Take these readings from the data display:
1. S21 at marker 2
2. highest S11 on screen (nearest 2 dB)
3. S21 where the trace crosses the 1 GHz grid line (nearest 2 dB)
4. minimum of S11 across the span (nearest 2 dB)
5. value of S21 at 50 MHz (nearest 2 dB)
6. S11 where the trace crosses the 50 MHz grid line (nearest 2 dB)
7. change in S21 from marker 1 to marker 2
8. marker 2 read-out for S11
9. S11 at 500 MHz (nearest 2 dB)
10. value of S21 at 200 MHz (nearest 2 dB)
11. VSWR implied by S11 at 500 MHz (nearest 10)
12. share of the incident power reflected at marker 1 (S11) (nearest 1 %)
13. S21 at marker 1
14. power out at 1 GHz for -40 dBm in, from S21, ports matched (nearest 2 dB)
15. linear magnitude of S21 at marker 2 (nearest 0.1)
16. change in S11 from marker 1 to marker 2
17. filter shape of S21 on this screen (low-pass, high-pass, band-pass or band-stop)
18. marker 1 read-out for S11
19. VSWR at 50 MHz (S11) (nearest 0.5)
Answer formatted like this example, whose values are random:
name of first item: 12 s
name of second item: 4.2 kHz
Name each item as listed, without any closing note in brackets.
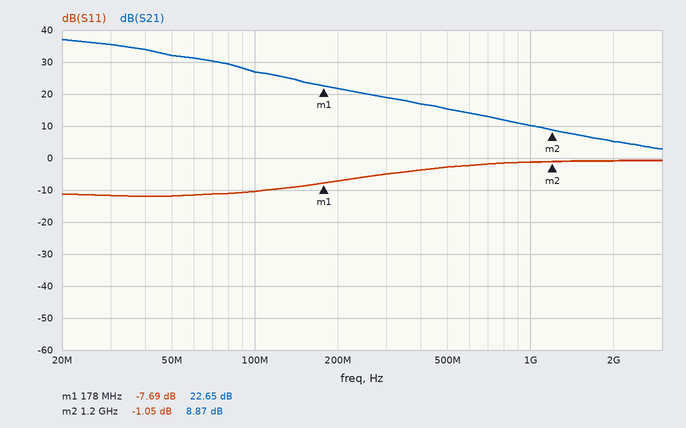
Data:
S21 at marker 2: 8.87 dB
highest S11 on screen: 0 dB
S21 where the trace crosses the 1 GHz grid line: 10 dB
minimum of S11 across the span: -12 dB
value of S21 at 50 MHz: 32 dB
S11 where the trace crosses the 50 MHz grid line: -12 dB
change in S21 from marker 1 to marker 2: -13.78 dB
marker 2 read-out for S11: -1.05 dB
S11 at 500 MHz: -2 dB
value of S21 at 200 MHz: 22 dB
VSWR implied by S11 at 500 MHz: 10
share of the incident power reflected at marker 1 (S11): 17 %
S21 at marker 1: 22.65 dB
power out at 1 GHz for -40 dBm in, from S21, ports matched: -30 dBm
linear magnitude of S21 at marker 2: 2.8
change in S11 from marker 1 to marker 2: 6.64 dB
filter shape of S21 on this screen: low-pass
marker 1 read-out for S11: -7.69 dB
VSWR at 50 MHz (S11): 1.5
